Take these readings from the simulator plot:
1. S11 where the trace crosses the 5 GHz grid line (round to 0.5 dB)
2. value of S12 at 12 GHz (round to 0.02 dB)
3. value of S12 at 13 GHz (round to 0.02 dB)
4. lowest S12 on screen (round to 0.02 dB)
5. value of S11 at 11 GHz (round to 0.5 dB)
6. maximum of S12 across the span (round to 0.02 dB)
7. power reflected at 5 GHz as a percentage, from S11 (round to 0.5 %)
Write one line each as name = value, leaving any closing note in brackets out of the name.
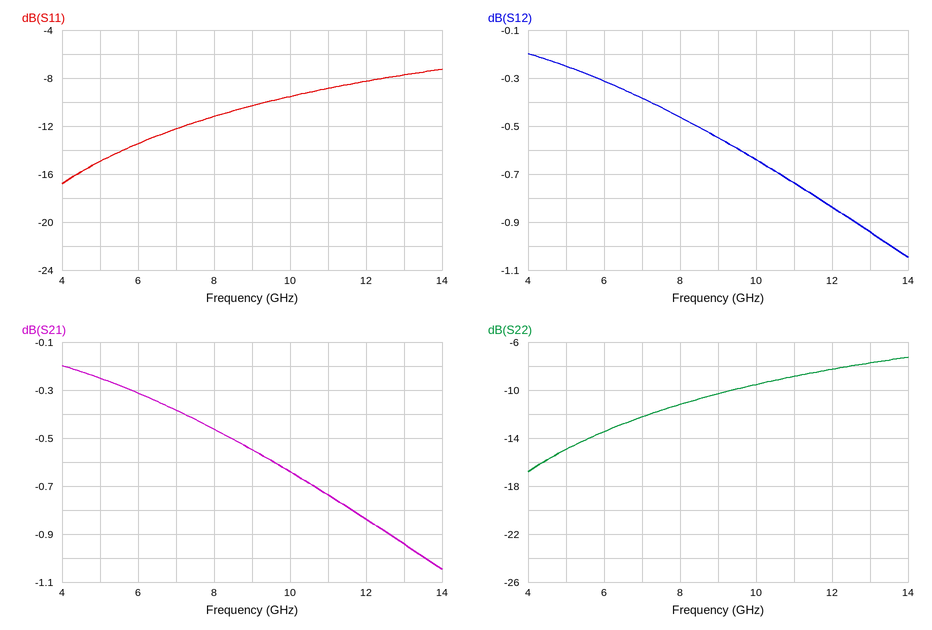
S11 where the trace crosses the 5 GHz grid line = -15.0 dB
value of S12 at 12 GHz = -0.84 dB
value of S12 at 13 GHz = -0.94 dB
lowest S12 on screen = -1.04 dB
value of S11 at 11 GHz = -9.0 dB
maximum of S12 across the span = -0.20 dB
power reflected at 5 GHz as a percentage, from S11 = 3.0 %
